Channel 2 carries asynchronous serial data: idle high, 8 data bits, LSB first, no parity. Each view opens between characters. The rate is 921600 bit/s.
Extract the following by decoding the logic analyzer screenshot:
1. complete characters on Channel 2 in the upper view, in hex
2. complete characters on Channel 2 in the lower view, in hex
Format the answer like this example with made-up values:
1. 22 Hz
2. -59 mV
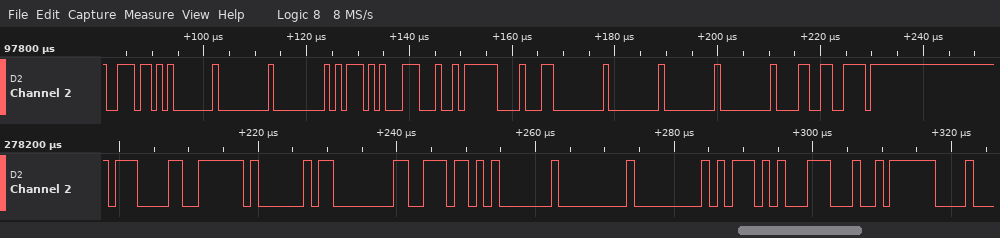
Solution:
1. 6E, 01, 00, 00, 5D, 1C, FA, 88, 00, 00, 00, 00, 98, DE
2. 87, 7E, A0, 80, 6E, 01, 00, 00, 5D, 1C, FA
